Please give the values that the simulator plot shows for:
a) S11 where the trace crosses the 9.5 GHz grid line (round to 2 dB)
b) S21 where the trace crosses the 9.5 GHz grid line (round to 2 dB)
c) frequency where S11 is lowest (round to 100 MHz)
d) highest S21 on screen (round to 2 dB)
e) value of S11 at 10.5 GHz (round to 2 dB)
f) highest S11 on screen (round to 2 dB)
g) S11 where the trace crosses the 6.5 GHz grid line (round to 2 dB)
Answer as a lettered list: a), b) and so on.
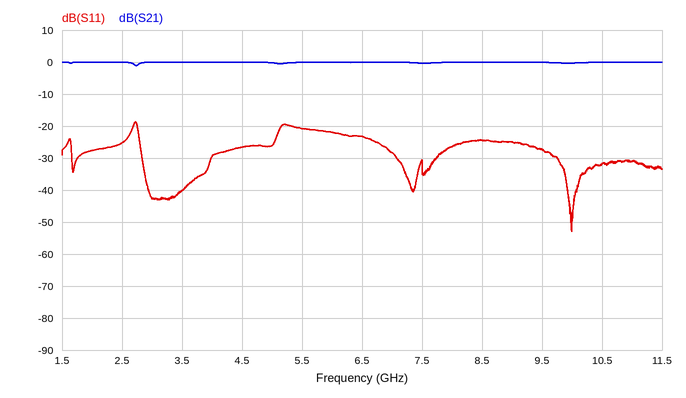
a) -28 dB
b) 0 dB
c) 10.0 GHz
d) 0 dB
e) -32 dB
f) -18 dB
g) -24 dB
